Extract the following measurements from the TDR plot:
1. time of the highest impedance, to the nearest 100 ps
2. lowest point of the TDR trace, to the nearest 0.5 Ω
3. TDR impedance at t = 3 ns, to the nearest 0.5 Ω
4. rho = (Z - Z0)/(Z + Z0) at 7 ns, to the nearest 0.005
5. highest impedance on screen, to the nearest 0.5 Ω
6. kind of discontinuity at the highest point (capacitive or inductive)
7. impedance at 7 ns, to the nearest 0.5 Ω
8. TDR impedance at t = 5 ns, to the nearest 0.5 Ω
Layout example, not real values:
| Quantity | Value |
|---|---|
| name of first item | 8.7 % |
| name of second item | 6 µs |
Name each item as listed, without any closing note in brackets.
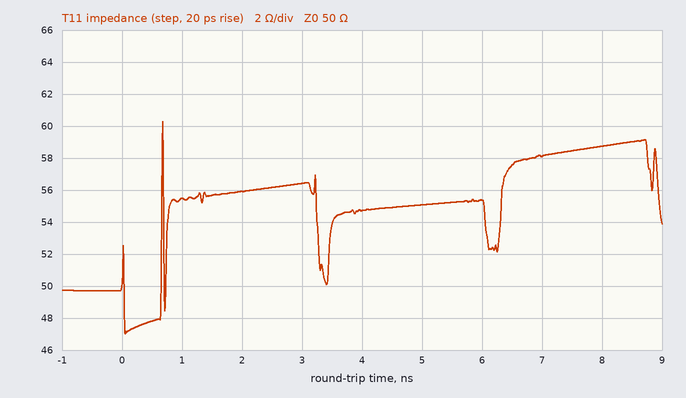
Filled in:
| Quantity | Value |
|---|---|
| time of the highest impedance, to the nearest 100 ps | 700 ps |
| lowest point of the TDR trace, to the nearest 0.5 Ω | 47.0 Ω |
| TDR impedance at t = 3 ns, to the nearest 0.5 Ω | 56.5 Ω |
| rho = (Z - Z0)/(Z + Z0) at 7 ns, to the nearest 0.005 | +0.075 |
| highest impedance on screen, to the nearest 0.5 Ω | 60.5 Ω |
| kind of discontinuity at the highest point | inductive |
| impedance at 7 ns, to the nearest 0.5 Ω | 58.0 Ω |
| TDR impedance at t = 5 ns, to the nearest 0.5 Ω | 55.0 Ω |
